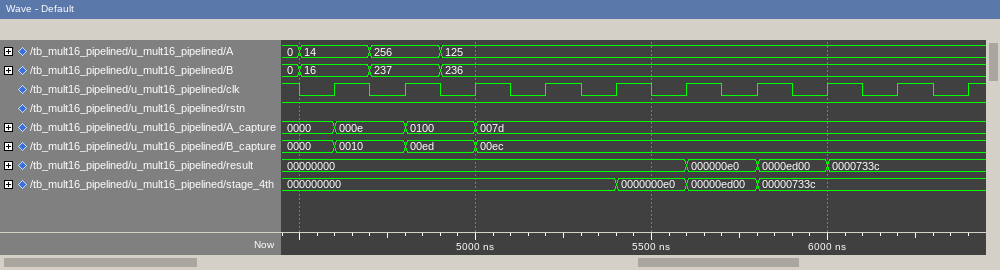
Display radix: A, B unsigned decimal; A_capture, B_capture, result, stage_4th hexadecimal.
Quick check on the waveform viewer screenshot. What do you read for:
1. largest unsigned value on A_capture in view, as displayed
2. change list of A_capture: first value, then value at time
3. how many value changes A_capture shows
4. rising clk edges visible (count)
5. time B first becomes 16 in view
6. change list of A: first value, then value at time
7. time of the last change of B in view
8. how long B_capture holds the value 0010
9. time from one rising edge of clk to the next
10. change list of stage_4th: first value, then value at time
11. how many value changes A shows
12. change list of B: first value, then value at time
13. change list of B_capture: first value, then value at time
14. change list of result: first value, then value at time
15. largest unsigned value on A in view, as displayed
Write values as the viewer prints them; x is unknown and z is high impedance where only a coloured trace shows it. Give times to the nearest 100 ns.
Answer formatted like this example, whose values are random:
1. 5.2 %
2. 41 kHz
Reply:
1. 0100
2. 0000, 000e at 4600 ns, 0100 at 4800 ns, 007d at 5000 ns
3. 3
4. 10
5. 4500 ns
6. 0, 14 at 4500 ns, 256 at 4700 ns, 125 at 4900 ns
7. 4900 ns
8. 200 ns
9. 200 ns
10. 000000000, 0000000e0 at 5400 ns, 00000ed00 at 5600 ns, 00000733c at 5800 ns
11. 3
12. 0, 16 at 4500 ns, 237 at 4700 ns, 236 at 4900 ns
13. 0000, 0010 at 4600 ns, 00ed at 4800 ns, 00ec at 5000 ns
14. 00000000, 000000e0 at 5600 ns, 0000ed00 at 5800 ns, 0000733c at 6000 ns
15. 256
